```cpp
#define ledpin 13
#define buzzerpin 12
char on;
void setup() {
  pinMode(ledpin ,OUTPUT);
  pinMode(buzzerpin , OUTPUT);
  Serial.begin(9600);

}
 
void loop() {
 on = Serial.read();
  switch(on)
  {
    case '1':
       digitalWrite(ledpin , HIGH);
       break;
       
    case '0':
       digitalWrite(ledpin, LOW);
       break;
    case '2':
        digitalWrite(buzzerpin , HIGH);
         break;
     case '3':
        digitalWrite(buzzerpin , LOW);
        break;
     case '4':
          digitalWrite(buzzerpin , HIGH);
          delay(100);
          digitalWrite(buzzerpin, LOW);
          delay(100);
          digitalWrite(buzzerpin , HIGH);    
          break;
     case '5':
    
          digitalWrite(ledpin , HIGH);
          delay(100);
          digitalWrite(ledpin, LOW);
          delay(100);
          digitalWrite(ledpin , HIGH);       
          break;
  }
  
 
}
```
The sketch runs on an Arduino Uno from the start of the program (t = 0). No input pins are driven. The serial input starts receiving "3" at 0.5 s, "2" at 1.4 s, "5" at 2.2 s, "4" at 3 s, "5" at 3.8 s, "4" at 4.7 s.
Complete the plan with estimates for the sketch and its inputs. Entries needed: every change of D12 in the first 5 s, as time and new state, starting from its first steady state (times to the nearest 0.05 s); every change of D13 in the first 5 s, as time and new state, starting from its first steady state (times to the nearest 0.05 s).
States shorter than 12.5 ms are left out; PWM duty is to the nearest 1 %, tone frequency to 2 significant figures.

0 s low; 1.4 s high; 3.1 s low; 3.2 s high; 4.8 s low; 4.9 s high
0 s low; 2.2 s high; 2.3 s low; 2.4 s high; 3.9 s low; 4 s high
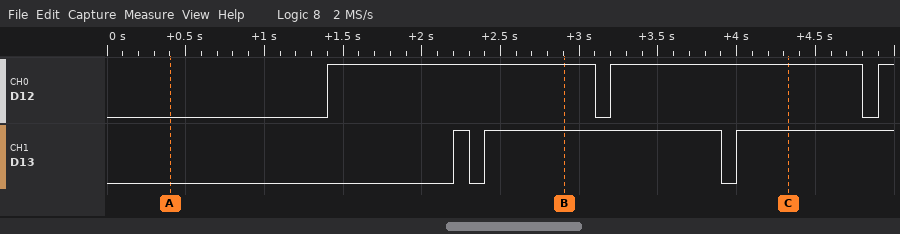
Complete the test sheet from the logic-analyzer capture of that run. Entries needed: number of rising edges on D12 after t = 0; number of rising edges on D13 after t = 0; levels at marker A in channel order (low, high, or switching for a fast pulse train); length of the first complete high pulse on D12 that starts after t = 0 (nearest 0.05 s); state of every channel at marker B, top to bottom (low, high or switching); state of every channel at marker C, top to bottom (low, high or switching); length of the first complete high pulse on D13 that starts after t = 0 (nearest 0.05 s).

3
3
D12 low, D13 low
1.70 s
D12 high, D13 high
D12 high, D13 high
0.10 s
